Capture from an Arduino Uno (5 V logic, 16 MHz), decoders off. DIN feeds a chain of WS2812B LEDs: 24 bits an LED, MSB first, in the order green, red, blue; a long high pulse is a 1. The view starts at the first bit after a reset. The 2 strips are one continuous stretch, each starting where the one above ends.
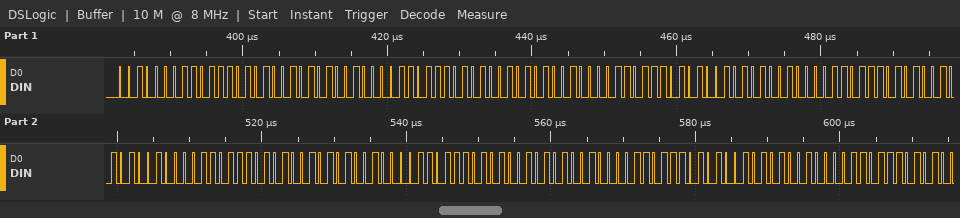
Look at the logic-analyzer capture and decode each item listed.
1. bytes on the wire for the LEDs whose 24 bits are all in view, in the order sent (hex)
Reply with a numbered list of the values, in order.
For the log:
1. 21 BA 95 21 BA 95 21 BA 95 21 BA 95 21 BA 95 21 BA 95 21 BA 95
